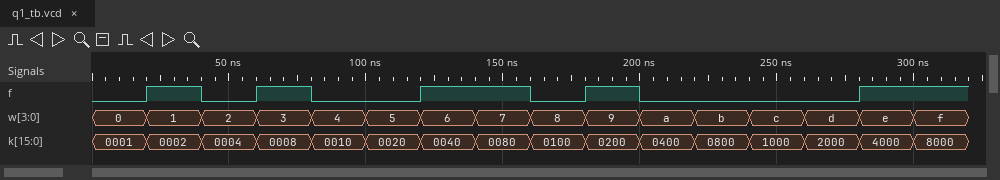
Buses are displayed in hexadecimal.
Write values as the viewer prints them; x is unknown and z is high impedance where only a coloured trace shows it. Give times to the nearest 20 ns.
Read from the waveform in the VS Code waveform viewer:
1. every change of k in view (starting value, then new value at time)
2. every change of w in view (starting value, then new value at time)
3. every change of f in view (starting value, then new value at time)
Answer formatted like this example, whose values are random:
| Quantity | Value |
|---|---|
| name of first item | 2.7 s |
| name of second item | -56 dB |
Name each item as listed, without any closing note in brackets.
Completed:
| Quantity | Value |
|---|---|
| every change of k in view | 0001, 0002 at 20 ns, 0004 at 40 ns, 0008 at 60 ns, 0010 at 80 ns, 0020 at 100 ns, 0040 at 120 ns, 0080 at 140 ns, 0100 at 160 ns, 0200 at 180 ns, 0400 at 200 ns, 0800 at 220 ns, 1000 at 240 ns, 2000 at 260 ns, 4000 at 280 ns, 8000 at 300 ns |
| every change of w in view | 0, 1 at 20 ns, 2 at 40 ns, 3 at 60 ns, 4 at 80 ns, 5 at 100 ns, 6 at 120 ns, 7 at 140 ns, 8 at 160 ns, 9 at 180 ns, a at 200 ns, b at 220 ns, c at 240 ns, d at 260 ns, e at 280 ns, f at 300 ns |
| every change of f in view | 0, 1 at 20 ns, 0 at 40 ns, 1 at 60 ns, 0 at 80 ns, 1 at 120 ns, 0 at 160 ns, 1 at 180 ns, 0 at 200 ns, 1 at 280 ns |
